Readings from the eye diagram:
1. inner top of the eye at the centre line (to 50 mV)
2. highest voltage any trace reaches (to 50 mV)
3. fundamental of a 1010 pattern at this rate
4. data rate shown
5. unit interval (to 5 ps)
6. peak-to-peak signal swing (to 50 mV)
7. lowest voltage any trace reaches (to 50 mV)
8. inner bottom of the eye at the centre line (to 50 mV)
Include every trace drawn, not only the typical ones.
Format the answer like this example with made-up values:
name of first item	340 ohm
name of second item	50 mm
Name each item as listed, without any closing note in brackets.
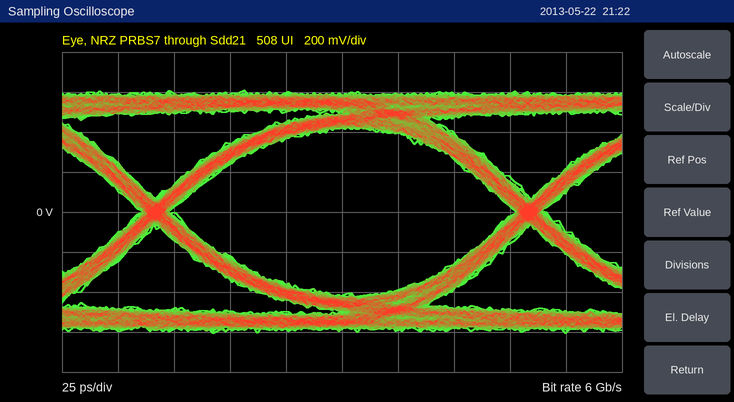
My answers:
inner top of the eye at the centre line	400 mV
highest voltage any trace reaches	600 mV
fundamental of a 1010 pattern at this rate	3 GHz
data rate shown	6 Gb/s
unit interval	165 ps
peak-to-peak signal swing	1.20 V
lowest voltage any trace reaches	-600 mV
inner bottom of the eye at the centre line	-400 mV
